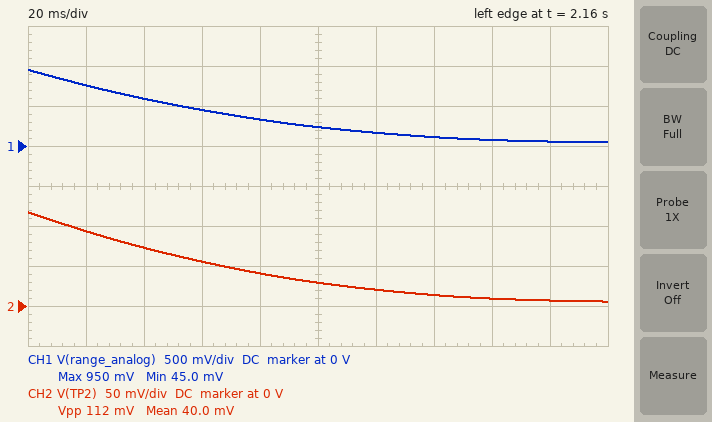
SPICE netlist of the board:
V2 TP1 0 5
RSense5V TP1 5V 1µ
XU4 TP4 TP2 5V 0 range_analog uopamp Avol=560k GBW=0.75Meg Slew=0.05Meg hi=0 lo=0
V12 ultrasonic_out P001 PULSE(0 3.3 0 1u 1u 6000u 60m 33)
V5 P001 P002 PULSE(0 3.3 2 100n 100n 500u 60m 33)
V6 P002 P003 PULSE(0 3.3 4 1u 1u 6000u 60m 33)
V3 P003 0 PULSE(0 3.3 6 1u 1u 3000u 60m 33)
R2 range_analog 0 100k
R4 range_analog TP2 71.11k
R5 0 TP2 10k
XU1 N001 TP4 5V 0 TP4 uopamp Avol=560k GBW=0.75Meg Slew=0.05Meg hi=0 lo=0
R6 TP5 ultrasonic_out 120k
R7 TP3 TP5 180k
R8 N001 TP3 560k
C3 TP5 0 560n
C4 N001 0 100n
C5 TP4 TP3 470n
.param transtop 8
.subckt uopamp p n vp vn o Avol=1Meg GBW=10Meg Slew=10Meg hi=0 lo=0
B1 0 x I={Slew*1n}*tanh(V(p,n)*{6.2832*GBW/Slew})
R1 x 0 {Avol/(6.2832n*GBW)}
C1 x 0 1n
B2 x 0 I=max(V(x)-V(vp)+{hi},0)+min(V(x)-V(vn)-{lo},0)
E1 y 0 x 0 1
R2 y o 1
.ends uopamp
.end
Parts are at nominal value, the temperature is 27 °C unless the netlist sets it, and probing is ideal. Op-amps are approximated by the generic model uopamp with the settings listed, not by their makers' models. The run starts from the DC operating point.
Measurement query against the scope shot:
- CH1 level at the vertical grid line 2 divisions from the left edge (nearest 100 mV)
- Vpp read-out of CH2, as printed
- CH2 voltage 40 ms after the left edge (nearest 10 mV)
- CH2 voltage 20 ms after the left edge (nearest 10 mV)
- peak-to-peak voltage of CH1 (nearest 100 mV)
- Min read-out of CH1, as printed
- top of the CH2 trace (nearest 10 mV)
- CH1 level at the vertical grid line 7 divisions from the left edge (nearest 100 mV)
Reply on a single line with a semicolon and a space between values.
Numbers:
600 mV; 112 mV; 70 mV; 90 mV; 900 mV; 45.0 mV; 120 mV; 100 mV
